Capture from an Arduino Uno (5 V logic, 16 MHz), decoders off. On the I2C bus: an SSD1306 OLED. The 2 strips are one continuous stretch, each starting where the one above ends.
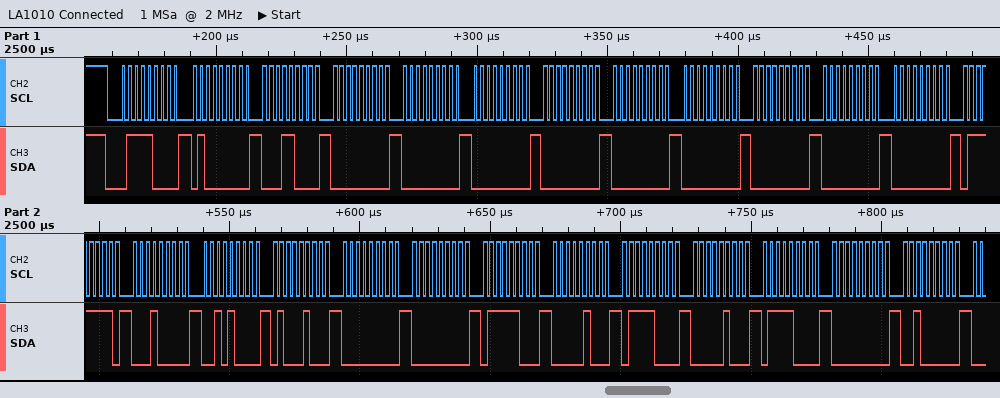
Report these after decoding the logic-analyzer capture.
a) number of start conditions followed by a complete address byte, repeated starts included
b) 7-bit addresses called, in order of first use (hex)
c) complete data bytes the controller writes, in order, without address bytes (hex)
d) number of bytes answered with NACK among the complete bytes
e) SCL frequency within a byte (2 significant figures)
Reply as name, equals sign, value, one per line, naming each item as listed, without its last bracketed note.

number of start conditions followed by a complete address byte, repeated starts included = 1
7-bit addresses called, in order of first use = 0x3C
complete data bytes the controller writes, in order, without address bytes = 40 18 00 00 00 00 00 00 00 00 00 7F 10 28 44 00 00 7C 04 78 04 78 00 20
number of bytes answered with NACK among the complete bytes = 0
SCL frequency within a byte = 400 kHz
